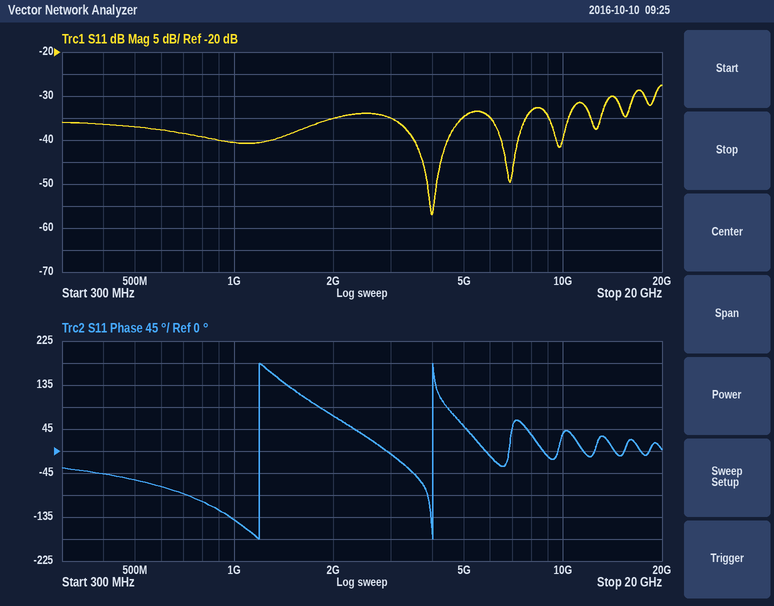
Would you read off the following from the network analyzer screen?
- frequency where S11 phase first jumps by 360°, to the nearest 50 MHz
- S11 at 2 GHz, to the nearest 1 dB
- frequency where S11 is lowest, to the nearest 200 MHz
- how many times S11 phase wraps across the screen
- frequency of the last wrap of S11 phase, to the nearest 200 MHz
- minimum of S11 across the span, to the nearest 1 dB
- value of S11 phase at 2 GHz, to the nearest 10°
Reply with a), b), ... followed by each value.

a) 1.20 GHz
b) -35 dB
c) 4.0 GHz
d) 2
e) 4.0 GHz
f) -57 dB
g) 70°
